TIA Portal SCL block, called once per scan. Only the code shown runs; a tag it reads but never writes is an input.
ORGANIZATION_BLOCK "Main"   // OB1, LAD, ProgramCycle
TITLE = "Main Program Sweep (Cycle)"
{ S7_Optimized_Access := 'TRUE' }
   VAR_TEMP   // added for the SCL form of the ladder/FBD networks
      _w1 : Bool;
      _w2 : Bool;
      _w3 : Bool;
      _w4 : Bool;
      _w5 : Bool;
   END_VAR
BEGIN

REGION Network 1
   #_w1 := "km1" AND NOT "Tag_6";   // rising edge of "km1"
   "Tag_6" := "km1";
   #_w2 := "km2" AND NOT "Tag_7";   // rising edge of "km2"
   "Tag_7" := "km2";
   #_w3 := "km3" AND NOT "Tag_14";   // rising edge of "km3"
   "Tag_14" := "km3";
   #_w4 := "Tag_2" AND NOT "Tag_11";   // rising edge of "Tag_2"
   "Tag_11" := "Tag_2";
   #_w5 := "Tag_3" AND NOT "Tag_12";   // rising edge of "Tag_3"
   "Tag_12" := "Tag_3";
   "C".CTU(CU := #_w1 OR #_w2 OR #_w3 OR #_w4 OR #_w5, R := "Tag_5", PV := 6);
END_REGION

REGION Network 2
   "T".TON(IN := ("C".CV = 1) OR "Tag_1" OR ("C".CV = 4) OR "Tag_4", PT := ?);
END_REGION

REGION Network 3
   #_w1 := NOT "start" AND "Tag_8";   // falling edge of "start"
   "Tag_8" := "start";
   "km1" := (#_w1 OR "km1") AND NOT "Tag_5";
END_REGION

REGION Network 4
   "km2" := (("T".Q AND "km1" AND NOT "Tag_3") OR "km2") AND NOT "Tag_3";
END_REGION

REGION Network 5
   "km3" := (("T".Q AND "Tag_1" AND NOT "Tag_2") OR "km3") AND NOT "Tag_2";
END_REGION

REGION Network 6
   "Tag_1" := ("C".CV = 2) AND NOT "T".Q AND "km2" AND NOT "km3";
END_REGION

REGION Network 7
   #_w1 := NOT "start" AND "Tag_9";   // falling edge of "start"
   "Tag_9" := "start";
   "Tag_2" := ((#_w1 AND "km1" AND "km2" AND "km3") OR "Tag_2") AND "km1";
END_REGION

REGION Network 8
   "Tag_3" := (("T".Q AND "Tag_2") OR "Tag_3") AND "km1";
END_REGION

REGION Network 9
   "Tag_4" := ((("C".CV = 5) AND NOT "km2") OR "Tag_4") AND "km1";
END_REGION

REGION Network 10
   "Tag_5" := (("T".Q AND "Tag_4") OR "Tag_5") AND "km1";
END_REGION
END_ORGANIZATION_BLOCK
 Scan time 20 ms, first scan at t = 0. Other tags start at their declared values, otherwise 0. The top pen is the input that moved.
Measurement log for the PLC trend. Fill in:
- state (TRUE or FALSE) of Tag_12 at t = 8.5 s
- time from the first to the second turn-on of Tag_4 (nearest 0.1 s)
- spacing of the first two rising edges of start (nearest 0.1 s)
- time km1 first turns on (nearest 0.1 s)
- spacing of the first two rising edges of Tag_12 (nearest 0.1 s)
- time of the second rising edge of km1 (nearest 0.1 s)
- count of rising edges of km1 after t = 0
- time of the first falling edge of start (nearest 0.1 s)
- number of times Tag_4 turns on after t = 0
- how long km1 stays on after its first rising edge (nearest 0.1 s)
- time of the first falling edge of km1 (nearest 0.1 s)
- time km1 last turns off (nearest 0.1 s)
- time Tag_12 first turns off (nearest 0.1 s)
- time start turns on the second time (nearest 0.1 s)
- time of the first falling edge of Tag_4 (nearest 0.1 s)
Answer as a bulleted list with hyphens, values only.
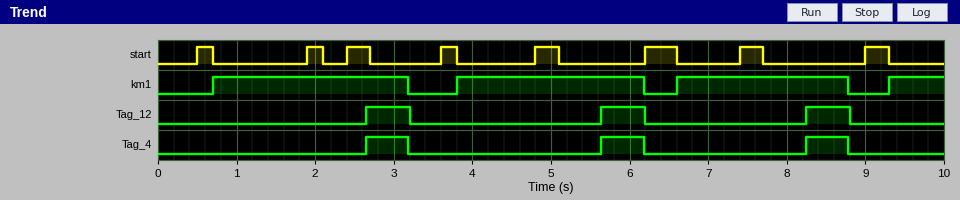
- TRUE
- 3.0 s
- 1.4 s
- 0.7 s
- 3.0 s
- 3.8 s
- 4
- 0.7 s
- 3
- 2.5 s
- 3.2 s
- 8.8 s
- 3.2 s
- 1.9 s
- 3.2 s
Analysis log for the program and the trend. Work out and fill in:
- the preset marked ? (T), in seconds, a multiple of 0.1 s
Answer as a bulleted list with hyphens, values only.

- 0.5 s
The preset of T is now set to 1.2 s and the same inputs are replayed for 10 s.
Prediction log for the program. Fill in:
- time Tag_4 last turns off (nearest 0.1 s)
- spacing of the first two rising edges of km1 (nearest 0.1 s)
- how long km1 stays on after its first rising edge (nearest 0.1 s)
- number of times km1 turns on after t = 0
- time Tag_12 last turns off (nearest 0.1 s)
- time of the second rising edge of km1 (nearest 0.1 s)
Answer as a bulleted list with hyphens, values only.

- 6.3 s
- 5.9 s
- 5.6 s
- 2
- 6.3 s
- 6.6 s
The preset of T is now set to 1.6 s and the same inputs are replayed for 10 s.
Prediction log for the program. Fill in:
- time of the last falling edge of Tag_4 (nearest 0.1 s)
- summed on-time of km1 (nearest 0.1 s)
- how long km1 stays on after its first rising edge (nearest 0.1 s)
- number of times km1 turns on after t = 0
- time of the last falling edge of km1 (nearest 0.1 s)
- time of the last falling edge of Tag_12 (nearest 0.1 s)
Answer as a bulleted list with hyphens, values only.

- 8.4 s
- 8.4 s
- 7.7 s
- 2
- 8.4 s
- 8.4 s
